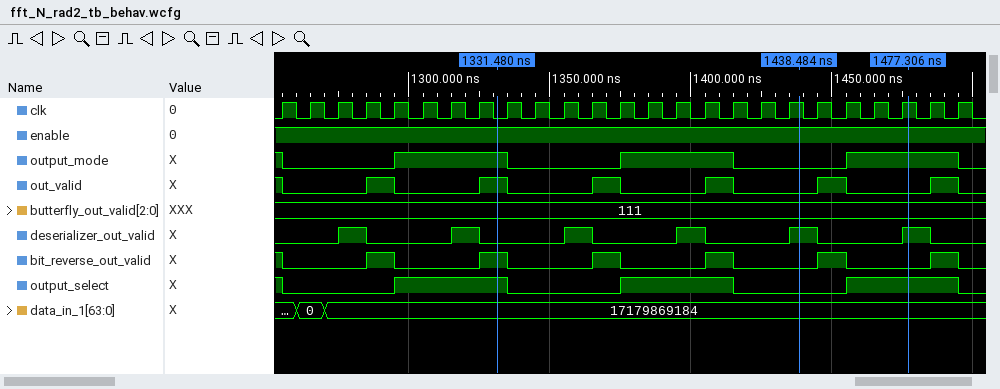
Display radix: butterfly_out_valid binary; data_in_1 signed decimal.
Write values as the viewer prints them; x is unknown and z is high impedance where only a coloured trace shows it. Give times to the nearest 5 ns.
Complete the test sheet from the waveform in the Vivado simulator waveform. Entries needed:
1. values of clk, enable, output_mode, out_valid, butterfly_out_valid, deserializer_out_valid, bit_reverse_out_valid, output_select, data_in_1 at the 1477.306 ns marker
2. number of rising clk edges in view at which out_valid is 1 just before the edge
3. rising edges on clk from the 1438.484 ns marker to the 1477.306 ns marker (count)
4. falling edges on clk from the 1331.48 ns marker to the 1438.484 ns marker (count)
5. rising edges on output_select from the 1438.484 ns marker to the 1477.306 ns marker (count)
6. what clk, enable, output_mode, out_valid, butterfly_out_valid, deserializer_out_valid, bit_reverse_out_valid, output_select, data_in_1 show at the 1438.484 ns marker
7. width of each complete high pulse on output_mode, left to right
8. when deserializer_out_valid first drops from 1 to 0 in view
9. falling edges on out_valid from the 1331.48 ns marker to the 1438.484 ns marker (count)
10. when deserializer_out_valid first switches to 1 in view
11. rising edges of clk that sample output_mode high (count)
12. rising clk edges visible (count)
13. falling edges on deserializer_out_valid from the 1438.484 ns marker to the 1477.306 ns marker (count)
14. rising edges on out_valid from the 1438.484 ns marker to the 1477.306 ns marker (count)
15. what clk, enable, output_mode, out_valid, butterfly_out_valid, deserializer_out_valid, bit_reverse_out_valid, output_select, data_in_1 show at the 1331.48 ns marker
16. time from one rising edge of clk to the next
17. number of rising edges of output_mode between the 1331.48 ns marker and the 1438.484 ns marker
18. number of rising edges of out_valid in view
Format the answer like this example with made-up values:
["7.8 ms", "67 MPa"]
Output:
["clk=1, enable=1, output_mode=1, out_valid=0, butterfly_out_valid=111, deserializer_out_valid=1, bit_reverse_out_valid=0, output_select=1, data_in_1=17179869184", "7", "4", "10", "1", "clk=1, enable=1, output_mode=0, out_valid=0, butterfly_out_valid=111, deserializer_out_valid=1, bit_reverse_out_valid=0, output_select=0, data_in_1=17179869184", "40 ns, 40 ns, 40 ns", "1285 ns", "3", "1275 ns", "13", "25", "1", "1", "clk=0, enable=1, output_mode=1, out_valid=1, butterfly_out_valid=111, deserializer_out_valid=0, bit_reverse_out_valid=1, output_select=1, data_in_1=17179869184", "10 ns", "1", "6"]
